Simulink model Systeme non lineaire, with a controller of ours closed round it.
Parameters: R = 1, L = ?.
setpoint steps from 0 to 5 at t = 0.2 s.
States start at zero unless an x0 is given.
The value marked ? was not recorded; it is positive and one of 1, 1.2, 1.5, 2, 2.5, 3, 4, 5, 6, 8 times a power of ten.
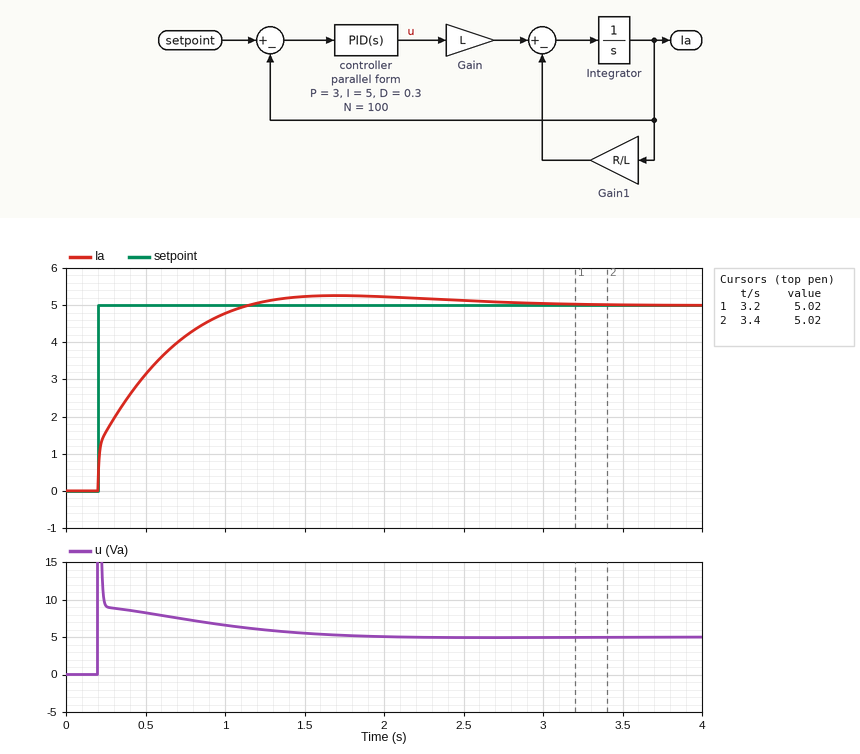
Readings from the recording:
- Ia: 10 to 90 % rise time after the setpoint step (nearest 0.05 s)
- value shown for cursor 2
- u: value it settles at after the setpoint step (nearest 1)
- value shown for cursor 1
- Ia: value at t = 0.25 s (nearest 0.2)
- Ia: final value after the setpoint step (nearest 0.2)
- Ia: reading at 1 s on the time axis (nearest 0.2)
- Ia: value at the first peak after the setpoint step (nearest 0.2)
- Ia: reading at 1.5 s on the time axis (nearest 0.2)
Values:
0.65 s
5.02
5
5.02
1.6
5.0
4.8
5.2
5.2
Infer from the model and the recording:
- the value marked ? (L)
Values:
1
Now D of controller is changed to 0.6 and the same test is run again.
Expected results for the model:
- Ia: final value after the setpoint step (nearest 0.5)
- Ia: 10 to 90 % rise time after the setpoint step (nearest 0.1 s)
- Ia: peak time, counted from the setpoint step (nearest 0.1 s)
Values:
5.0
0.8 s
1.7 s
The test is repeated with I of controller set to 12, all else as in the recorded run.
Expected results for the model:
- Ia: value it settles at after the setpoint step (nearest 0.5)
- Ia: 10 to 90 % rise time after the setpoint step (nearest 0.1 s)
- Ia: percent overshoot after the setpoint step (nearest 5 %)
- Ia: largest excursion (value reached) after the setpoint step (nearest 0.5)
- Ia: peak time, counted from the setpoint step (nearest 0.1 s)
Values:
5.0
0.4 s
15 %
6.0
0.9 s
